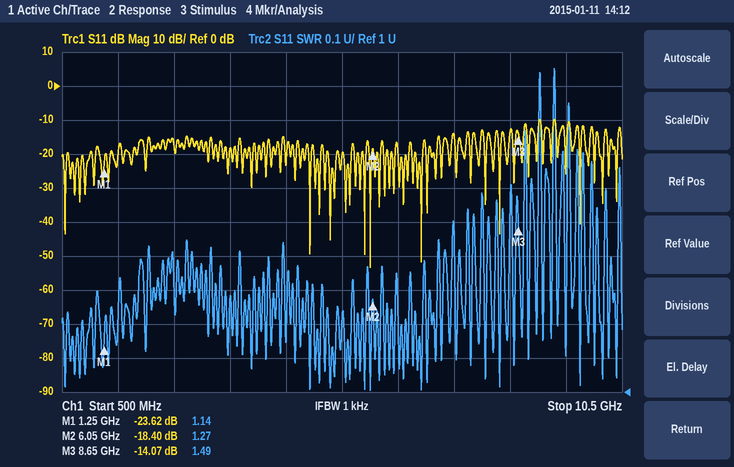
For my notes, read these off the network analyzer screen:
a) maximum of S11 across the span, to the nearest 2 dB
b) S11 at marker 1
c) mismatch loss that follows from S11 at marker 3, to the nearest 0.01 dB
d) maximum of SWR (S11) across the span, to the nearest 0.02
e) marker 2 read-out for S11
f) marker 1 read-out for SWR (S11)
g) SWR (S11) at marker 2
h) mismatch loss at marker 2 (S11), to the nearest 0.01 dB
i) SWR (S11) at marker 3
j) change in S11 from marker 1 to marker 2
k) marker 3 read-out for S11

-10 dB
-23.62 dB
0.17 dB
1.96
-18.40 dB
1.14
1.27
0.06 dB
1.49
5.22 dB
-14.07 dB
